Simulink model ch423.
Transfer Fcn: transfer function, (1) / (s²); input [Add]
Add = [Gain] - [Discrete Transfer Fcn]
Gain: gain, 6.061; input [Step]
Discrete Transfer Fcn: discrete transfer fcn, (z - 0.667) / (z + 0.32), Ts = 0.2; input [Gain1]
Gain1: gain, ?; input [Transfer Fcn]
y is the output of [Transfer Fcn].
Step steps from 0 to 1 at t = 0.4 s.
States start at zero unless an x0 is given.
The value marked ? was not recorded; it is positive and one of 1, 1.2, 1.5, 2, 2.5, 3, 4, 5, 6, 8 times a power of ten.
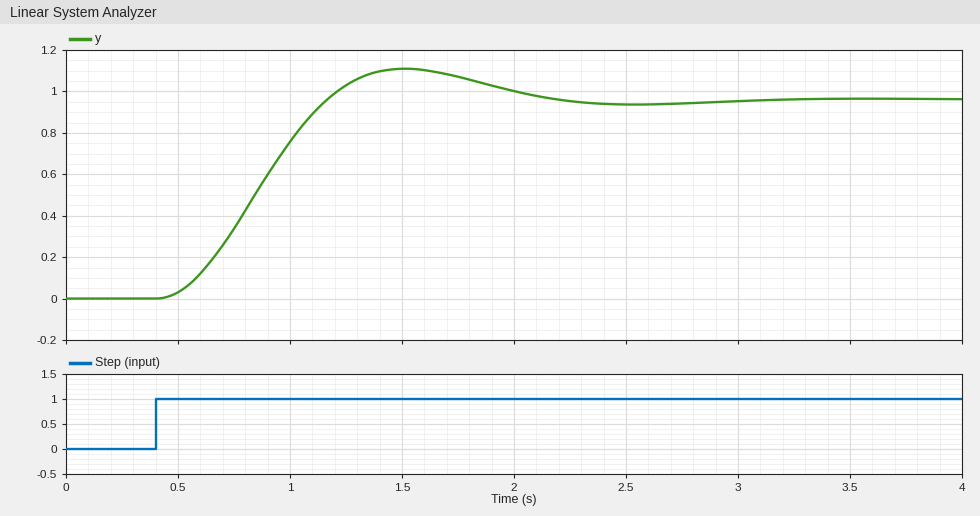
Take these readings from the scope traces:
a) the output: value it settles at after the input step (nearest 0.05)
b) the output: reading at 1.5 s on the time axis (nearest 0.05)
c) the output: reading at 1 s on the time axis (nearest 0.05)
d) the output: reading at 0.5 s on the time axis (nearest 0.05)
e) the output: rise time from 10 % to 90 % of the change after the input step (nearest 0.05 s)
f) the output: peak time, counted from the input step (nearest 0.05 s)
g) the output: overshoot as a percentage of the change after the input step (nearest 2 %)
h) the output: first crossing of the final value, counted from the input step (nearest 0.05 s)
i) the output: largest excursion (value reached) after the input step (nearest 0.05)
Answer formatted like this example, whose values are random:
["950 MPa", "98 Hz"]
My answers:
["0.95", "1.10", "0.75", "0.05", "0.50 s", "1.10 s", "16 %", "0.75 s", "1.10"]
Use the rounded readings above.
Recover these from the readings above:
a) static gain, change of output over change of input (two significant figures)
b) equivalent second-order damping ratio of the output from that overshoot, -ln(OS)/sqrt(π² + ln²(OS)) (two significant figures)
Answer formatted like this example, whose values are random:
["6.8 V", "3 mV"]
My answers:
["0.95", "0.50"]
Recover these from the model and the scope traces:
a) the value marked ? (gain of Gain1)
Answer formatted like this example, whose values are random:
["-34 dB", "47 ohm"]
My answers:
["25"]
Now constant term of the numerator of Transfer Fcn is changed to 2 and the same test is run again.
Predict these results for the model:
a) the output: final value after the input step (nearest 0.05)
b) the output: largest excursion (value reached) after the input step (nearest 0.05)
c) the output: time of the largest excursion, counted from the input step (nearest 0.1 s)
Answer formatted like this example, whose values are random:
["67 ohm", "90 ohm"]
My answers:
["0.95", "1.00", "1.4 s"]
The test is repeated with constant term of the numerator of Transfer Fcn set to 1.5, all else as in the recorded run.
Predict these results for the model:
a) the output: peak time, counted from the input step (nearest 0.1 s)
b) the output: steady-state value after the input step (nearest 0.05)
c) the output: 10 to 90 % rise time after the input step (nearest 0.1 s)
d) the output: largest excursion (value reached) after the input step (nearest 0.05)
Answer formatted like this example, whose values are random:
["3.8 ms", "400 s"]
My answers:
["0.8 s", "0.95", "0.4 s", "1.00"]
